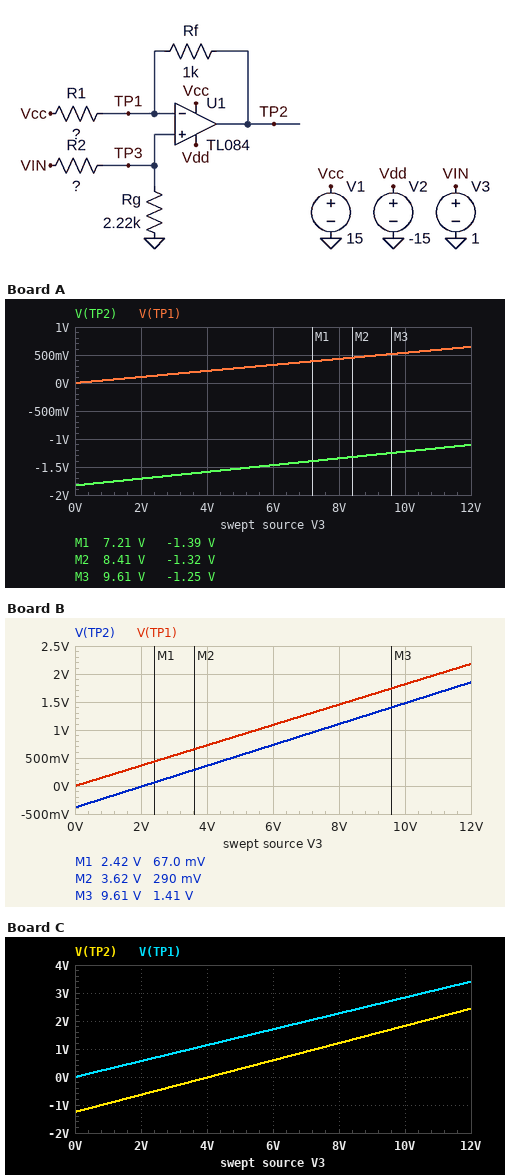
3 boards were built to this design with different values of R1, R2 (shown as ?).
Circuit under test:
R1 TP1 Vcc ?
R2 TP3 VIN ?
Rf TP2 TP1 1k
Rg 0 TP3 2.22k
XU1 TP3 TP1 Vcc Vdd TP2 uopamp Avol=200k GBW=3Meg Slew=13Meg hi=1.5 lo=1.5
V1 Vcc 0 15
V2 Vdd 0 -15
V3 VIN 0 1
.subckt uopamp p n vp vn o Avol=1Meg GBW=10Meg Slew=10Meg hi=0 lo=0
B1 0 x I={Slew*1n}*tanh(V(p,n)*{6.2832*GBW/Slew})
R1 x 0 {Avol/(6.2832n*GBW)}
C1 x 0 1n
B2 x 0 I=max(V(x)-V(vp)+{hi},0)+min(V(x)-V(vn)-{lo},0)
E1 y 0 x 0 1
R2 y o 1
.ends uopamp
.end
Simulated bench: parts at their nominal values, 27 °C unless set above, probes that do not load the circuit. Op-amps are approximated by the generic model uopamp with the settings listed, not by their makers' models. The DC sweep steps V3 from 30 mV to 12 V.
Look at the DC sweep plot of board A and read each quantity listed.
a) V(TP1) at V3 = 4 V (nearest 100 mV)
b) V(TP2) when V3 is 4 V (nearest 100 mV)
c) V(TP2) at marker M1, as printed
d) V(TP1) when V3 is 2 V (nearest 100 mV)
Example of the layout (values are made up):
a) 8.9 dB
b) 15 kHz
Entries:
a) 200 mV
b) -1.6 V
c) -1.39 V
d) 100 mV
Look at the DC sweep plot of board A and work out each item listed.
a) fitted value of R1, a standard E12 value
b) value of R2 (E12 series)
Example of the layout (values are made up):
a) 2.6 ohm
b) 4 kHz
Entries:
a) 8.2 kΩ
b) 39 kΩ
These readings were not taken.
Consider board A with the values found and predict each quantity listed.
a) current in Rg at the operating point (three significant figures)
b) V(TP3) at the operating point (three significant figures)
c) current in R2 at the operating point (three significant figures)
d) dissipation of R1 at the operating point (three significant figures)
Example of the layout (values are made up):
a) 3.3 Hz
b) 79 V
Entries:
a) 24.3 µA
b) 53.9 mV
c) 24.3 µA
d) 27.2 mW
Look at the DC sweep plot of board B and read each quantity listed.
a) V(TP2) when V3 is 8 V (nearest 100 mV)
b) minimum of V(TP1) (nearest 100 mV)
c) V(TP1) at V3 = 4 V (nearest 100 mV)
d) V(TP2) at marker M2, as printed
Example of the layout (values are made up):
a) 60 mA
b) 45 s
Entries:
a) 1.1 V
b) 0 V
c) 700 mV
d) 290 mV
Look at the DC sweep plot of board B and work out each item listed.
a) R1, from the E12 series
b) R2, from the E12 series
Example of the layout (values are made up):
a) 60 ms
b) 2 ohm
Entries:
a) 39 kΩ
b) 10 kΩ
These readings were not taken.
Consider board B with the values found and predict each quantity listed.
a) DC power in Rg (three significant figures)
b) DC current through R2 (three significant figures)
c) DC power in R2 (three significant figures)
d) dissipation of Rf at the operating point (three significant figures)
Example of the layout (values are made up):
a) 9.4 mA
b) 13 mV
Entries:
a) 14.9 µW
b) 81.8 µA
c) 67.0 µW
d) 144 µW
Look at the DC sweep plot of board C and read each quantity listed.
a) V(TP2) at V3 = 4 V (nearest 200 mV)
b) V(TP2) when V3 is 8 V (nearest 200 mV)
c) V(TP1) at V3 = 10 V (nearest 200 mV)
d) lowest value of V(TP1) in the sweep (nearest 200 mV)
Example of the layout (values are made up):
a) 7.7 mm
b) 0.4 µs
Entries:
a) 0 V
b) 1.2 V
c) 2.8 V
d) 0 V
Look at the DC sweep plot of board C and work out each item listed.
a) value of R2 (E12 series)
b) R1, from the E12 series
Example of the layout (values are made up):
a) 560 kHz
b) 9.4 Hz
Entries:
a) 5.6 kΩ
b) 12 kΩ
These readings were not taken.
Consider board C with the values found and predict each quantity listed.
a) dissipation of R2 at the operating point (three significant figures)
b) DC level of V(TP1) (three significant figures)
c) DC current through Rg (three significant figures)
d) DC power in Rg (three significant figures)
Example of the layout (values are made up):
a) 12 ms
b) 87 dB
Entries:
a) 91.6 µW
b) 284 mV
c) 128 µA
d) 36.3 µW
